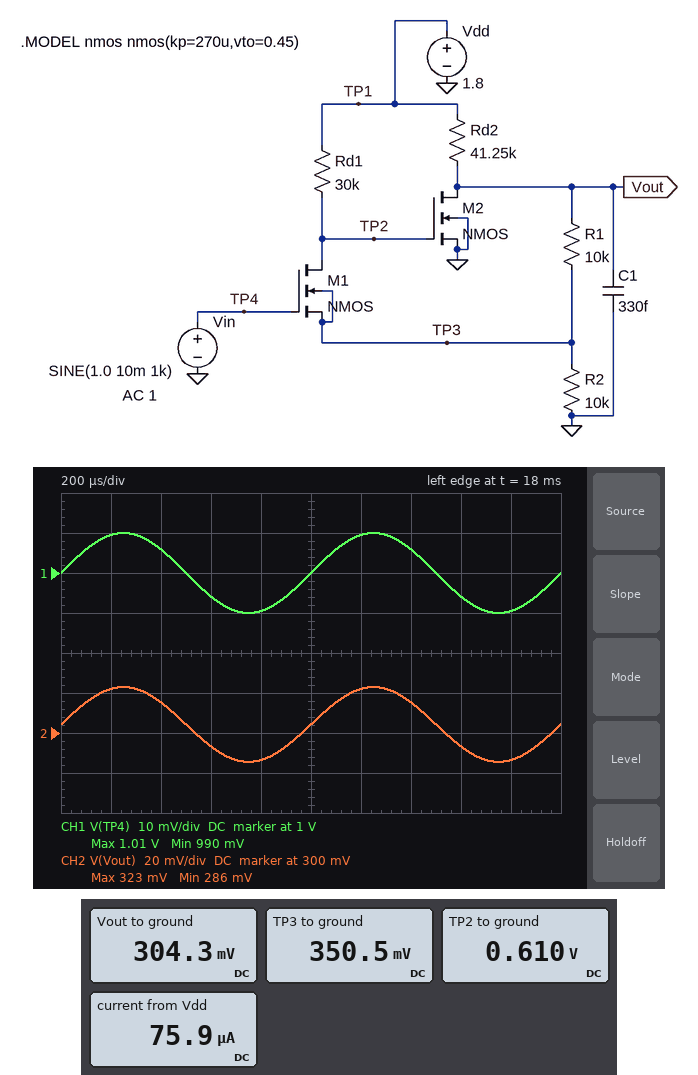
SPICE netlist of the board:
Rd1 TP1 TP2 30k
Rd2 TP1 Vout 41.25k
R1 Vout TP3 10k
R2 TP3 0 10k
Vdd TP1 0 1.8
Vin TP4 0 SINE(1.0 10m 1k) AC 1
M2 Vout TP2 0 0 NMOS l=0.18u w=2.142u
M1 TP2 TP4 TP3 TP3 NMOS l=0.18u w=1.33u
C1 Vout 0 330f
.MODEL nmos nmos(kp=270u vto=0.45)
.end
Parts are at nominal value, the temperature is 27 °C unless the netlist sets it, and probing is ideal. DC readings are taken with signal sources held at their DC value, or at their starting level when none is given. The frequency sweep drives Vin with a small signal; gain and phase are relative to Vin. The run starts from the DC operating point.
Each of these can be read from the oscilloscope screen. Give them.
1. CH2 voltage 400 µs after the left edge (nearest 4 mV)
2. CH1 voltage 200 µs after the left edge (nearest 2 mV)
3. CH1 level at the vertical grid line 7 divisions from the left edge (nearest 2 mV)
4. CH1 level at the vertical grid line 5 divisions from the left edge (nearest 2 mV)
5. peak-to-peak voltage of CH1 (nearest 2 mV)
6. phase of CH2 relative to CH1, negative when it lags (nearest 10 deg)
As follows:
316 mV
1.010 V
1.006 V
1.000 V
20 mV
0 deg
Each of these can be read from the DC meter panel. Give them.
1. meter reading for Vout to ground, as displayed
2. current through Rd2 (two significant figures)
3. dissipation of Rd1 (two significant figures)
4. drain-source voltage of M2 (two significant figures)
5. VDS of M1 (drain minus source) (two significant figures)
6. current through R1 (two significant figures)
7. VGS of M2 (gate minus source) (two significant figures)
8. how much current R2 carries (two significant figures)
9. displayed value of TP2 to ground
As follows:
304.3 mV
36 µA
47 µW
300 mV
260 mV
4.6 µA
610 mV
35 µA
0.610 V
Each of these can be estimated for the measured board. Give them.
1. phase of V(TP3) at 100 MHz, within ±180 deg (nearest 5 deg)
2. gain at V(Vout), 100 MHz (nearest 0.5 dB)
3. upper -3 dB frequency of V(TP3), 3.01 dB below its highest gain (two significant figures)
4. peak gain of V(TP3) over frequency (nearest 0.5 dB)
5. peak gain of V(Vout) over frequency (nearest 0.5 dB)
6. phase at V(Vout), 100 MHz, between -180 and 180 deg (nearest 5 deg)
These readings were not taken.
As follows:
-5 deg
5.5 dB
2.0 GHz
0 dB
5.5 dB
-10 deg
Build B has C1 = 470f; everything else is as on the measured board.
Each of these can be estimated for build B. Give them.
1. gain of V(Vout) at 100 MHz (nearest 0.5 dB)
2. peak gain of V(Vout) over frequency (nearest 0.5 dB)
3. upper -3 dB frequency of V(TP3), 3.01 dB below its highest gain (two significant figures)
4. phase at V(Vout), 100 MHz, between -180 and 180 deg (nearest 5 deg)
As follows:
5.0 dB
5.5 dB
1.4 GHz
-15 deg
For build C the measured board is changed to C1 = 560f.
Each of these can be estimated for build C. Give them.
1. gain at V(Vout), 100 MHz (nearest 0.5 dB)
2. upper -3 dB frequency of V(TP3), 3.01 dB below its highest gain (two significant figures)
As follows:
5.0 dB
1.2 GHz
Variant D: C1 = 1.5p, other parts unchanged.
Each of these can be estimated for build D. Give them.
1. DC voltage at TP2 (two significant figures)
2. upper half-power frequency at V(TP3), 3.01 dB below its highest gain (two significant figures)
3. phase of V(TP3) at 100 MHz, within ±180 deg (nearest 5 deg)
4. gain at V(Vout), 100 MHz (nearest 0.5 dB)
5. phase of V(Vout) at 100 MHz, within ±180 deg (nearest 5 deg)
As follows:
610 mV
440 MHz
-10 deg
3.0 dB
-40 deg
